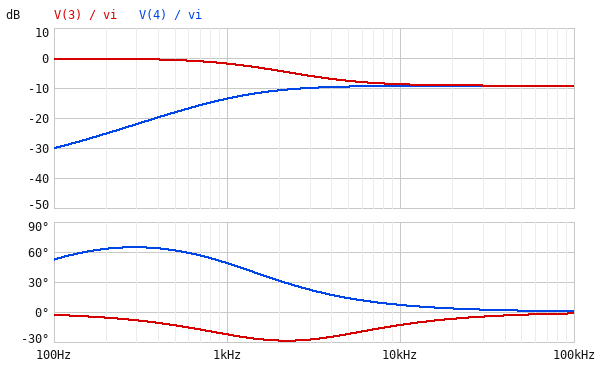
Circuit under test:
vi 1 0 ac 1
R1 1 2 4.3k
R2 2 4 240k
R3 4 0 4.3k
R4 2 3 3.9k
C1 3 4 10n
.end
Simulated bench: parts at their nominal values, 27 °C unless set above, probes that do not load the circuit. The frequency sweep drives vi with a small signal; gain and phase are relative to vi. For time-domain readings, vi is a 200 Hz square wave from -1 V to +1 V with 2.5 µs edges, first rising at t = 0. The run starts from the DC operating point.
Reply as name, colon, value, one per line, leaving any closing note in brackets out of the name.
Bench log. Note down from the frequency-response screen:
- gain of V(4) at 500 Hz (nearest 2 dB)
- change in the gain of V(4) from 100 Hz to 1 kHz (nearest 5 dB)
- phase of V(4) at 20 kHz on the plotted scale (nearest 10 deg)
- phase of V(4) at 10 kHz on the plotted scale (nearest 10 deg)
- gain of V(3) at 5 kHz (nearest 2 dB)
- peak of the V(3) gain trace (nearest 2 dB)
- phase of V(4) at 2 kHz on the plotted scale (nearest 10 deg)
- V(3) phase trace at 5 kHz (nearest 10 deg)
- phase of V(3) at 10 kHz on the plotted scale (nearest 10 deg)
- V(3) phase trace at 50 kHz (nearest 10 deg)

gain of V(4) at 500 Hz: -18 dB
change in the gain of V(4) from 100 Hz to 1 kHz: 15 dB
phase of V(4) at 20 kHz on the plotted scale: 0 deg
phase of V(4) at 10 kHz on the plotted scale: 10 deg
gain of V(3) at 5 kHz: -8 dB
peak of the V(3) gain trace: 0 dB
phase of V(4) at 2 kHz on the plotted scale: 30 deg
V(3) phase trace at 5 kHz: -20 deg
phase of V(3) at 10 kHz on the plotted scale: -10 deg
V(3) phase trace at 50 kHz: 0 deg
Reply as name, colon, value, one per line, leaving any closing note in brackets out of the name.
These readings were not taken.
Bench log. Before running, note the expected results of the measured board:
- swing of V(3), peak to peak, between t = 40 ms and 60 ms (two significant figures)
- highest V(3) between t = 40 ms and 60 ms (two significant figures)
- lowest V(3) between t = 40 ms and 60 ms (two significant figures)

swing of V(3), peak to peak, between t = 40 ms and 60 ms: 2.0 V
highest V(3) between t = 40 ms and 60 ms: 980 mV
lowest V(3) between t = 40 ms and 60 ms: -980 mV
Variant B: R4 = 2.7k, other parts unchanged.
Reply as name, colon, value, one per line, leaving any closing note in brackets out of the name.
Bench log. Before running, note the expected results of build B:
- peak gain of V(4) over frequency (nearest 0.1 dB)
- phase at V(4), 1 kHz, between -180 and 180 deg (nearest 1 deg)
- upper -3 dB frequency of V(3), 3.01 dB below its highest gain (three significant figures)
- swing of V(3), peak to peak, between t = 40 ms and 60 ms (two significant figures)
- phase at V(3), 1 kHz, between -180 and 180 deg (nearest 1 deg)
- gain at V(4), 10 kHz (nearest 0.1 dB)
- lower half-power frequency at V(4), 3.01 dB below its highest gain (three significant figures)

peak gain of V(4) over frequency: -8.4 dB
phase at V(4), 1 kHz, between -180 and 180 deg: 52 deg
upper -3 dB frequency of V(3), 3.01 dB below its highest gain: 1.73 kHz
swing of V(3), peak to peak, between t = 40 ms and 60 ms: 2.0 V
phase at V(3), 1 kHz, between -180 and 180 deg: -20 deg
gain at V(4), 10 kHz: -8.5 dB
lower half-power frequency at V(4), 3.01 dB below its highest gain: 1.44 kHz
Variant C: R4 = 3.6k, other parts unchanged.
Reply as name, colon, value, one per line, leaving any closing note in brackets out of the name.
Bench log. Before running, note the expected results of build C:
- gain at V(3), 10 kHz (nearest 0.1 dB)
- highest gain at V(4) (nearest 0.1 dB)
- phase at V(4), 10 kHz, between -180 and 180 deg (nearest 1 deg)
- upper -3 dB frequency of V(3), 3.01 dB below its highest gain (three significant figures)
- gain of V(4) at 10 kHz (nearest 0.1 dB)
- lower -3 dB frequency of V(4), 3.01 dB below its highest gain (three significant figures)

gain at V(3), 10 kHz: -8.5 dB
highest gain at V(4): -9.0 dB
phase at V(4), 10 kHz, between -180 and 180 deg: 7 deg
upper -3 dB frequency of V(3), 3.01 dB below its highest gain: 1.55 kHz
gain of V(4) at 10 kHz: -9.1 dB
lower -3 dB frequency of V(4), 3.01 dB below its highest gain: 1.33 kHz
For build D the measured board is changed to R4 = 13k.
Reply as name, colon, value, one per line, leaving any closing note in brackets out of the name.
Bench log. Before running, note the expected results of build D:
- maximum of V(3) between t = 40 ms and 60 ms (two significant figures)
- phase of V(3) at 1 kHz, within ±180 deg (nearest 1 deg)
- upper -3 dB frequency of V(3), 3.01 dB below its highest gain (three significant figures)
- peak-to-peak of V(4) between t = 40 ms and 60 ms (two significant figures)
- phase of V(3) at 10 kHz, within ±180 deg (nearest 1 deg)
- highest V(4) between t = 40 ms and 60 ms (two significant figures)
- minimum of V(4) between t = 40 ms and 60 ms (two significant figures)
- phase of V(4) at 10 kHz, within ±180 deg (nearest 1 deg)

maximum of V(3) between t = 40 ms and 60 ms: 980 mV
phase of V(3) at 1 kHz, within ±180 deg: -38 deg
upper -3 dB frequency of V(3), 3.01 dB below its highest gain: 782 Hz
peak-to-peak of V(4) between t = 40 ms and 60 ms: 780 mV
phase of V(3) at 10 kHz, within ±180 deg: -15 deg
highest V(4) between t = 40 ms and 60 ms: 390 mV
minimum of V(4) between t = 40 ms and 60 ms: -390 mV
phase of V(4) at 10 kHz, within ±180 deg: 4 deg
